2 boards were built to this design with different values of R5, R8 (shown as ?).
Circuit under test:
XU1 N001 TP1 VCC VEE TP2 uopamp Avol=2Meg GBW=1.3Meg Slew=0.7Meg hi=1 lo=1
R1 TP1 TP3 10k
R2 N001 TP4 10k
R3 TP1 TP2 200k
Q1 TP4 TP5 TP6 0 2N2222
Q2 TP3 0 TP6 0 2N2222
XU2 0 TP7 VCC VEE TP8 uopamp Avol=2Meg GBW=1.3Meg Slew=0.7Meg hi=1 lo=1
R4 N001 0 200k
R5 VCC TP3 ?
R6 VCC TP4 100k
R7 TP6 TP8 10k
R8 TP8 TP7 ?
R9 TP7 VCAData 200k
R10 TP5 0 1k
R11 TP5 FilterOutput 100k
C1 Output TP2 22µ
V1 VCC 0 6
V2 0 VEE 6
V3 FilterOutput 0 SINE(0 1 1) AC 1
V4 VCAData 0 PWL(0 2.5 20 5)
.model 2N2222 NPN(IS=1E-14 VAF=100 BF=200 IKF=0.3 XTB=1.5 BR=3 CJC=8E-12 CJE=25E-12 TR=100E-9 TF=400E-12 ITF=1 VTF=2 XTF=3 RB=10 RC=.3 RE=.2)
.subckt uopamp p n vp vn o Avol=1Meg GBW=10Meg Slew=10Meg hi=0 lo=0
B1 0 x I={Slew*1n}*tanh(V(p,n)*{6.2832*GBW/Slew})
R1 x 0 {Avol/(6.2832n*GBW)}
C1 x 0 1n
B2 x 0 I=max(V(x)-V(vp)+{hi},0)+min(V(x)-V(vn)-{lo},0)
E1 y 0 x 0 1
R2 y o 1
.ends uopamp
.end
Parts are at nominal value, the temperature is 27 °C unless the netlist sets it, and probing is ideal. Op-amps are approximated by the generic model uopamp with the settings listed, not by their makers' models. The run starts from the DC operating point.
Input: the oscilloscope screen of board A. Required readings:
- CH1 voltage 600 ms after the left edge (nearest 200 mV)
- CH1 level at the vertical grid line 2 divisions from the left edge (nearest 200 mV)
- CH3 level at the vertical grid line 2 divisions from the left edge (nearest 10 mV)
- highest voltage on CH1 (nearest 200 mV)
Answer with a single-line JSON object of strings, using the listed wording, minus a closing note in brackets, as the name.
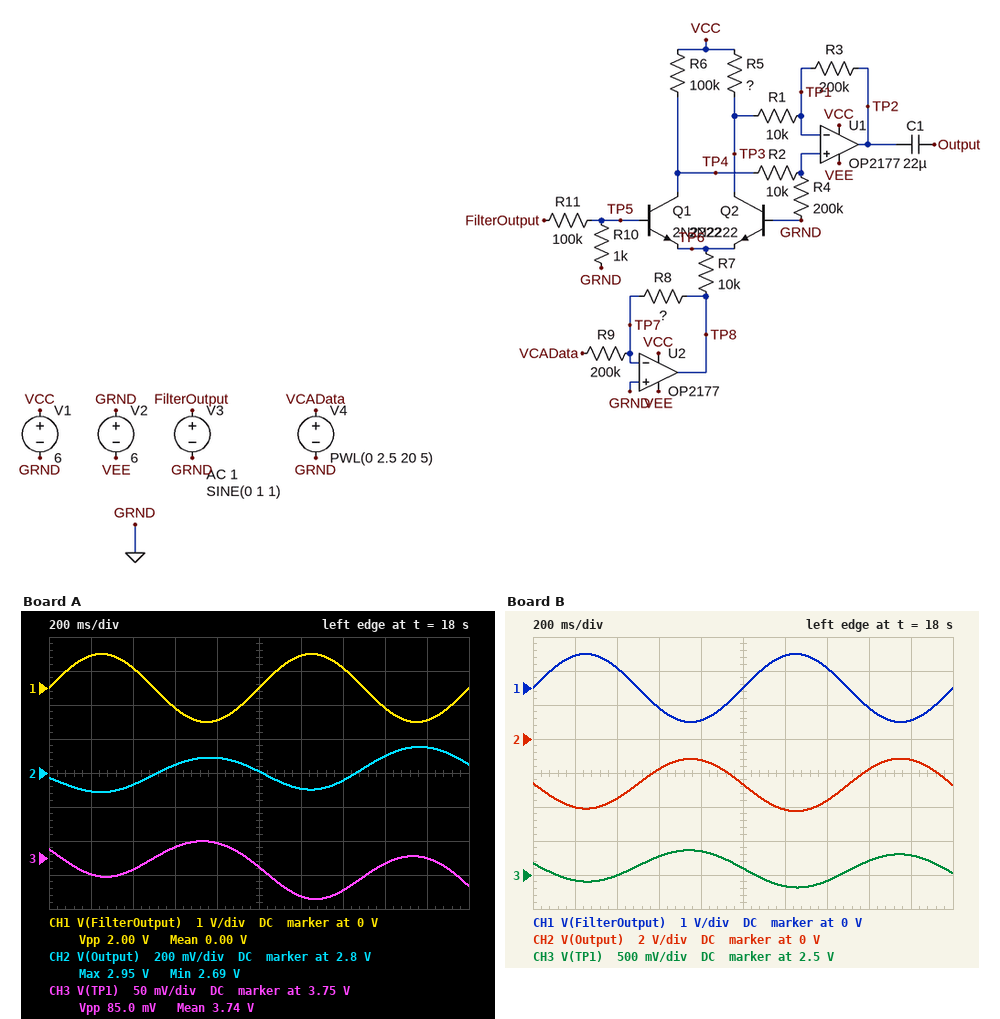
{"CH1 voltage 600 ms after the left edge": "-600 mV", "CH1 level at the vertical grid line 2 divisions from the left edge": "600 mV", "CH3 level at the vertical grid line 2 divisions from the left edge": "3.73 V", "highest voltage on CH1": "1.0 V"}
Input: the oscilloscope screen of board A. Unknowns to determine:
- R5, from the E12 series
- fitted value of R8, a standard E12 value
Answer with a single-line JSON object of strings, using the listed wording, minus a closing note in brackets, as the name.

{"R5, from the E12 series": "330 kΩ", "fitted value of R8, a standard E12 value": "22 kΩ"}
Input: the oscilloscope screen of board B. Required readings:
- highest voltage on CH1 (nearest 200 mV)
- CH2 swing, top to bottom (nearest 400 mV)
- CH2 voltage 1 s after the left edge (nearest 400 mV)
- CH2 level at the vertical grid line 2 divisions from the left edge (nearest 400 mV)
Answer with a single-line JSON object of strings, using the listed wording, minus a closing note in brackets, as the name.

{"highest voltage on CH1": "1.0 V", "CH2 swing, top to bottom": "3.2 V", "CH2 voltage 1 s after the left edge": "-2.8 V", "CH2 level at the vertical grid line 2 divisions from the left edge": "-3.6 V"}
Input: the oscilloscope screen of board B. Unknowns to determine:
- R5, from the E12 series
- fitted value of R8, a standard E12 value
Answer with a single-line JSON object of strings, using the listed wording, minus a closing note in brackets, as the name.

{"R5, from the E12 series": "68 kΩ", "fitted value of R8, a standard E12 value": "39 kΩ"}
